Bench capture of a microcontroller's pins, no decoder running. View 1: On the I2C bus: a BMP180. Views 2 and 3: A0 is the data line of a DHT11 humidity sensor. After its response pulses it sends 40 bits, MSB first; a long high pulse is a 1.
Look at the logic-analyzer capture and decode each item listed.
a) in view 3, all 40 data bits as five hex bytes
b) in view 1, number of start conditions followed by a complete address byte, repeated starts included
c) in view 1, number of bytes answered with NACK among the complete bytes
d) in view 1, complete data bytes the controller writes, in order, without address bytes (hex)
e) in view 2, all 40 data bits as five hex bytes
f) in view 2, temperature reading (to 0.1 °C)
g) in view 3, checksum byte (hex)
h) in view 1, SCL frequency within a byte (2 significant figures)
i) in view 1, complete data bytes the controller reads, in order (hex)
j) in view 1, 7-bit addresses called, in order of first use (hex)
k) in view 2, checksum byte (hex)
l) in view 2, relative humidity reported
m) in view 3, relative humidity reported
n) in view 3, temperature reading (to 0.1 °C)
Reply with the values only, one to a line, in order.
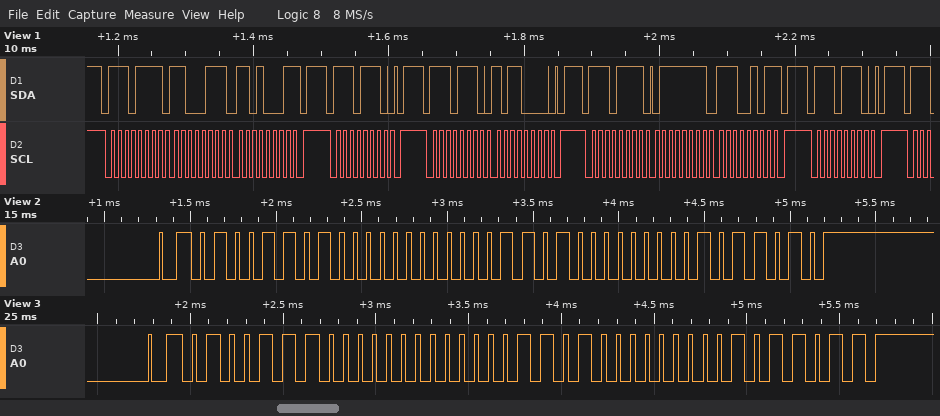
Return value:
4E 00 0D 00 5B
5
2
B0
4D 00 0D 00 5A
13.0 °C
0x5B
100 kHz
C7 D1 7F E5
0x77
0x5A
77 %
78 %
13.0 °C
